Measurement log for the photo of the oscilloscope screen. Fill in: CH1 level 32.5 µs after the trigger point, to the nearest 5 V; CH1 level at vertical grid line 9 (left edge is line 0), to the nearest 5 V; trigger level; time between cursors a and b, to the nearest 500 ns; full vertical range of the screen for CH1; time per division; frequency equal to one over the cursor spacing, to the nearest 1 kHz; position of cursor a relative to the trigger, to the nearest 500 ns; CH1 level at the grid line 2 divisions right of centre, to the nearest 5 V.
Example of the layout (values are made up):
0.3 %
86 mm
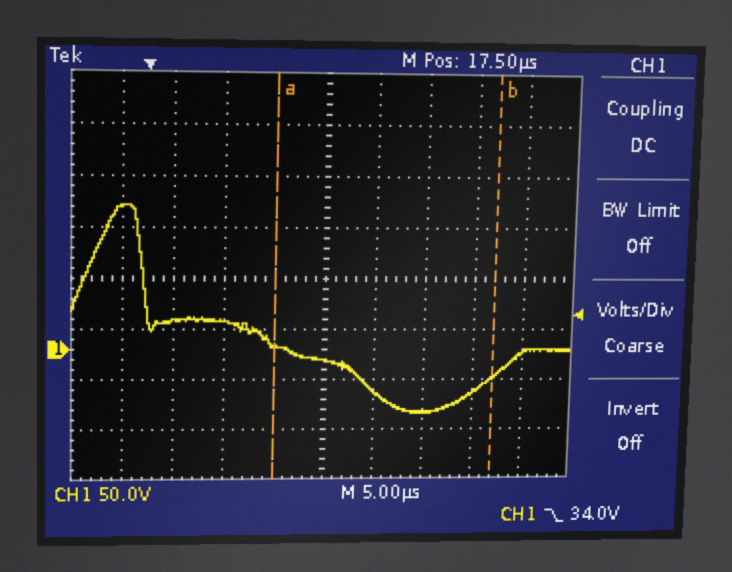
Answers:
-45 V
-5 V
34.0 V
22.0 µs
400 V
5 µs
45 kHz
+12.5 µs
-65 V
